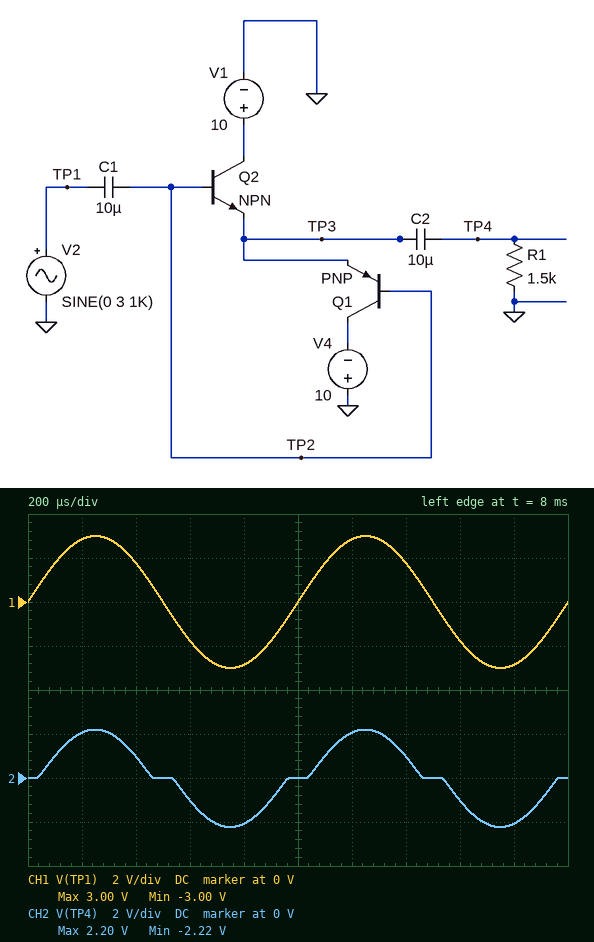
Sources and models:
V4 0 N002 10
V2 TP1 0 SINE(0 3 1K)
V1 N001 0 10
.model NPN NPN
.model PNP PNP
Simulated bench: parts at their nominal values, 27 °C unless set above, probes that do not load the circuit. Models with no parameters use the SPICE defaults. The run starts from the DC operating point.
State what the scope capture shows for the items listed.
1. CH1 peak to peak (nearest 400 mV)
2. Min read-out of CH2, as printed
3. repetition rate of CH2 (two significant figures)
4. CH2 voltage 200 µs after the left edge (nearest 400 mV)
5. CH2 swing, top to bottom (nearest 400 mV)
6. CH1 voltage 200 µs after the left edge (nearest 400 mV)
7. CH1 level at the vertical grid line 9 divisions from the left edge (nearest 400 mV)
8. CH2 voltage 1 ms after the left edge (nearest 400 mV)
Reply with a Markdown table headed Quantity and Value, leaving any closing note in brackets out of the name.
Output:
| Quantity | Value |
|---|---|
| CH1 peak to peak | 6.0 V |
| Min read-out of CH2, as printed | -2.22 V |
| repetition rate of CH2 | 1.0 kHz |
| CH2 voltage 200 µs after the left edge | 2.0 V |
| CH2 swing, top to bottom | 4.4 V |
| CH1 voltage 200 µs after the left edge | 2.8 V |
| CH1 level at the vertical grid line 9 divisions from the left edge | -2.8 V |
| CH2 voltage 1 ms after the left edge | 0 V |
